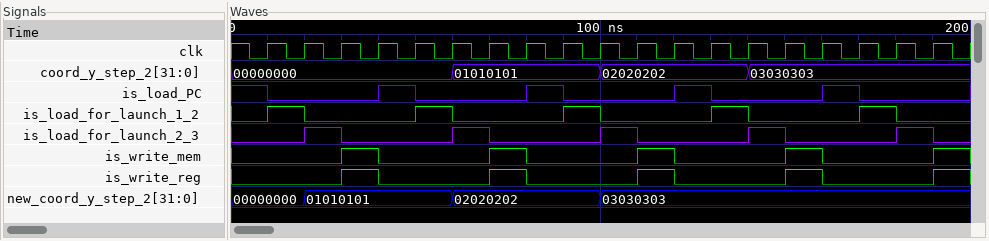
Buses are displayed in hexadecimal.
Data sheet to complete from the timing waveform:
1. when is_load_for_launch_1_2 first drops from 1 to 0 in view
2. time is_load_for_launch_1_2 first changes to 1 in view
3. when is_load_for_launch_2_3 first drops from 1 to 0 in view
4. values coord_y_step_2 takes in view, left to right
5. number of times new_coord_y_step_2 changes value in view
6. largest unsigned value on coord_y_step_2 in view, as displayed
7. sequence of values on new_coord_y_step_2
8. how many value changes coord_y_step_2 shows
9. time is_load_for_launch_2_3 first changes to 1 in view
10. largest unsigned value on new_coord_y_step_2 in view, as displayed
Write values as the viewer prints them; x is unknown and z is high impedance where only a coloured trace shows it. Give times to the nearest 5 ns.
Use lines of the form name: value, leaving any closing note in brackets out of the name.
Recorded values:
when is_load_for_launch_1_2 first drops from 1 to 0 in view: 20 ns
time is_load_for_launch_1_2 first changes to 1 in view: 10 ns
when is_load_for_launch_2_3 first drops from 1 to 0 in view: 30 ns
values coord_y_step_2 takes in view, left to right: 00000000, 01010101, 02020202, 03030303
number of times new_coord_y_step_2 changes value in view: 3
largest unsigned value on coord_y_step_2 in view, as displayed: 03030303
sequence of values on new_coord_y_step_2: 00000000, 01010101, 02020202, 03030303
how many value changes coord_y_step_2 shows: 3
time is_load_for_launch_2_3 first changes to 1 in view: 20 ns
largest unsigned value on new_coord_y_step_2 in view, as displayed: 03030303
